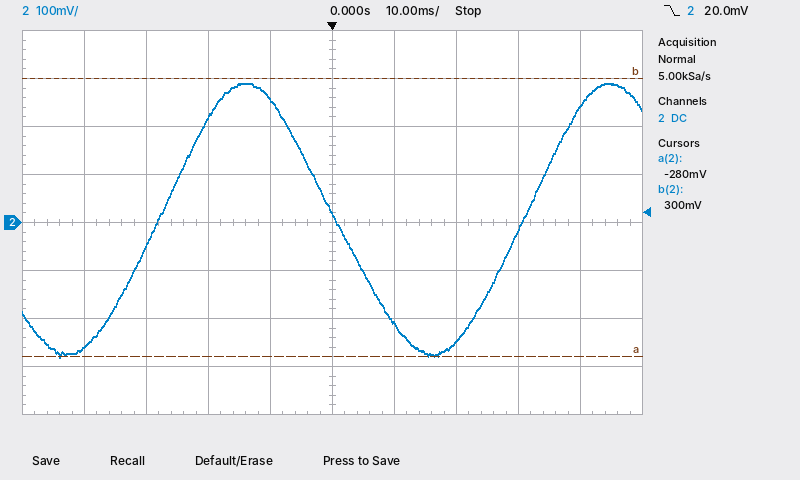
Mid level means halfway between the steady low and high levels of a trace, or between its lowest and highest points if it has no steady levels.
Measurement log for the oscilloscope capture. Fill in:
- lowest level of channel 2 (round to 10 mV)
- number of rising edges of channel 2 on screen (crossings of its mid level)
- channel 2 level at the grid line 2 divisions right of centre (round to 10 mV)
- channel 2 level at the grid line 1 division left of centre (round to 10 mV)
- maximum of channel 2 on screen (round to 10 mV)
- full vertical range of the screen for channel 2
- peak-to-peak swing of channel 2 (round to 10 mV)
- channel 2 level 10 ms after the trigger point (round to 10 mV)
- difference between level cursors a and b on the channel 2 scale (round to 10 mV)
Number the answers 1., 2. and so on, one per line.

1. -280 mV
2. 2
3. -250 mV
4. 260 mV
5. 290 mV
6. 800 mV
7. 570 mV
8. -210 mV
9. 580 mV
